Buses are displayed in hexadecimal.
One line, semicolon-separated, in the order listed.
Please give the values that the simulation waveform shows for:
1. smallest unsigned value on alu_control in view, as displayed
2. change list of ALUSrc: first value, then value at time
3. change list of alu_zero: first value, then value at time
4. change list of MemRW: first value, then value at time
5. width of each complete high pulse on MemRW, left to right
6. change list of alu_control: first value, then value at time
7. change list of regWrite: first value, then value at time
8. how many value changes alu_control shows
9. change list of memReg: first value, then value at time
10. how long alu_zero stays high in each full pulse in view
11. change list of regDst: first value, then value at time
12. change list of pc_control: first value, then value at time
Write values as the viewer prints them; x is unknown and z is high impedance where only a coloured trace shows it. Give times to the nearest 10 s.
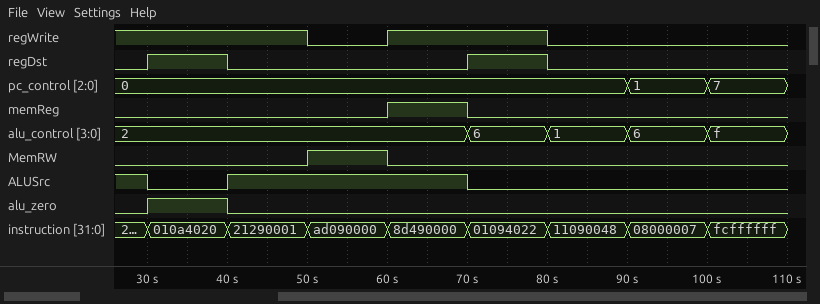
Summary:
1; 1, 0 at 30 s, 1 at 40 s, 0 at 70 s; 0, 1 at 30 s, 0 at 40 s; 0, 1 at 50 s, 0 at 60 s; 10 s; 2, 6 at 70 s, 1 at 80 s, 6 at 90 s, f at 100 s; 1, 0 at 50 s, 1 at 60 s, 0 at 80 s; 4; 0, 1 at 60 s, 0 at 70 s; 10 s; 0, 1 at 30 s, 0 at 40 s, 1 at 70 s, 0 at 80 s; 0, 1 at 90 s, 7 at 100 s
